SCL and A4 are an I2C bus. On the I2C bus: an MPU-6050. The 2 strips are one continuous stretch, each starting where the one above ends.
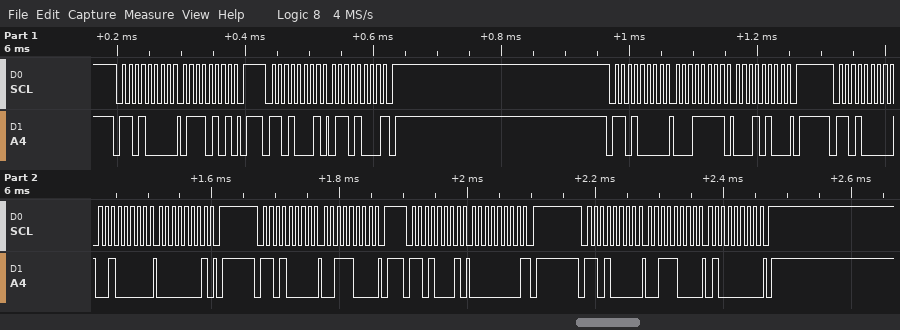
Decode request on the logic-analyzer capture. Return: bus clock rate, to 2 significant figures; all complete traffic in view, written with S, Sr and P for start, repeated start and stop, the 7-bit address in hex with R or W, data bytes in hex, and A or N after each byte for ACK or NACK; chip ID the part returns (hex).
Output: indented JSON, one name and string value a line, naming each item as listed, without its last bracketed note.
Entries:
{
  "bus clock rate, to 2 significant figures": "100 kHz",
  "all complete traffic in view, written with S, Sr and P for start, repeated start and stop, the 7-bit address in hex with R or W, data bytes in hex, and A or N after each byte for ACK or NACK": "S 68W A 75 A P S 68R A 68 N P S 68W A 1F A 14 A P S 68W A 20 A 01 A P S 68W A 38 A P S 68R A 00 N P S 68W A 38 A 40 A P",
  "chip ID the part returns": "0x68"
}
